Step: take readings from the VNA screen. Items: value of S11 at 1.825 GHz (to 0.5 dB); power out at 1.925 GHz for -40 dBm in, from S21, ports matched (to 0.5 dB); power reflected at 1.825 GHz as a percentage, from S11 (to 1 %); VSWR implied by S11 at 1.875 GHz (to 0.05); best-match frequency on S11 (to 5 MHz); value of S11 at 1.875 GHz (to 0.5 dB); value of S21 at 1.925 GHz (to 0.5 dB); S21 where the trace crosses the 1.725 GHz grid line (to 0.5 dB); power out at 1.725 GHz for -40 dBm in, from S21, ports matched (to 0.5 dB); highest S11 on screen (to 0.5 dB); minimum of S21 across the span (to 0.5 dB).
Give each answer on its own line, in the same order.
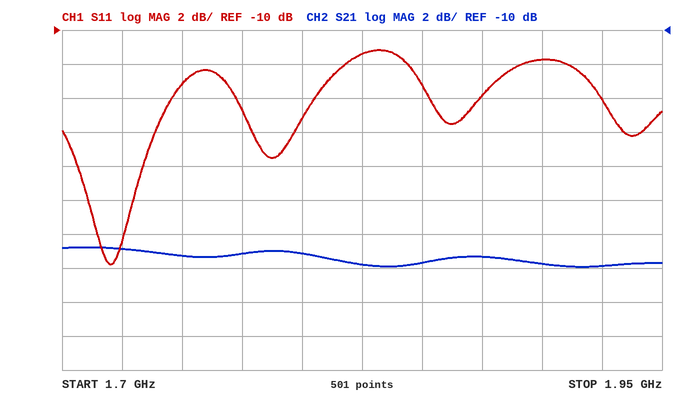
-11.5 dB
-64.0 dBm
7 %
1.50
1.720 GHz
-14.0 dB
-24.0 dB
-23.0 dB
-63.0 dBm
-11.0 dB
-24.0 dB
